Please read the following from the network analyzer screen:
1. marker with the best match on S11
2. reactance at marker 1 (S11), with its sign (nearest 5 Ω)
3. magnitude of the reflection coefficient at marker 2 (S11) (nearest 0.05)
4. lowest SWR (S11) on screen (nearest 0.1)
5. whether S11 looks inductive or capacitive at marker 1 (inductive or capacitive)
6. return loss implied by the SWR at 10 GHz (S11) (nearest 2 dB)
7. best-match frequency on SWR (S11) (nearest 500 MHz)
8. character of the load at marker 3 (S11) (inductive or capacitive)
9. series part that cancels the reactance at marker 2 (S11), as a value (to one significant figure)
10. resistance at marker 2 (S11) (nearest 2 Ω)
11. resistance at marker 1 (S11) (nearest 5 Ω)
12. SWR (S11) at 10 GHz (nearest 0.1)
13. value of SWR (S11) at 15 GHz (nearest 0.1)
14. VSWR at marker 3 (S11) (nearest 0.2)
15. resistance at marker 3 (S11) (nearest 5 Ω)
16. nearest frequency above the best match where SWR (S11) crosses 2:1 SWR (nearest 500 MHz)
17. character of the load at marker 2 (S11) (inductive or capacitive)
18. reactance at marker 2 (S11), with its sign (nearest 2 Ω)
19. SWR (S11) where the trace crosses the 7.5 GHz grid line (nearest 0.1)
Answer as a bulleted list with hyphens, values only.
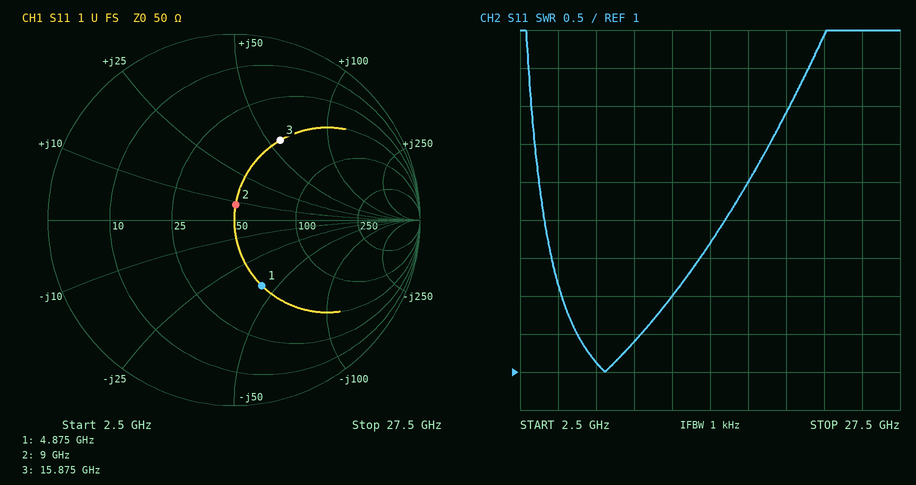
- marker 2
- -40 Ω
- 0.10
- 1.0
- capacitive
- 16 dB
- 8.0 GHz
- inductive
- 2 pF
- 50 Ω
- 50 Ω
- 1.4
- 2.7
- 3.0
- 50 Ω
- 12.5 GHz
- inductive
- +8 Ω
- 1.1
